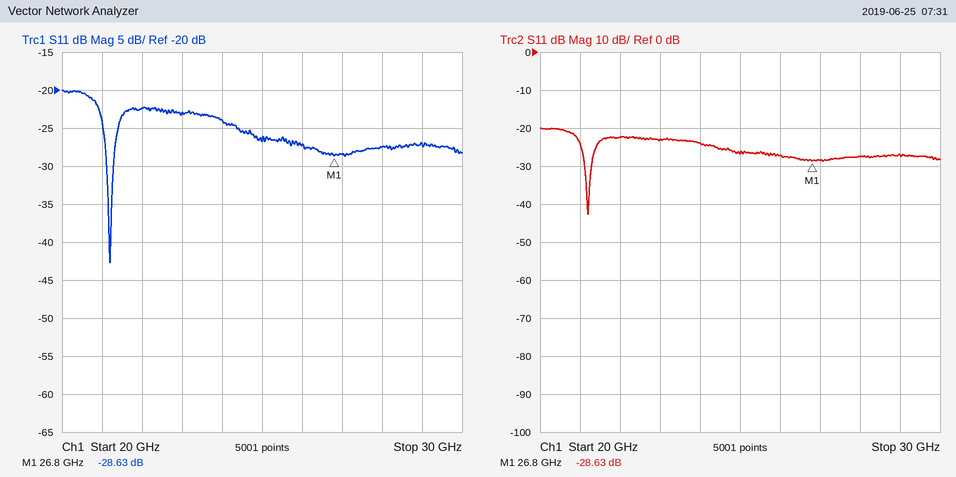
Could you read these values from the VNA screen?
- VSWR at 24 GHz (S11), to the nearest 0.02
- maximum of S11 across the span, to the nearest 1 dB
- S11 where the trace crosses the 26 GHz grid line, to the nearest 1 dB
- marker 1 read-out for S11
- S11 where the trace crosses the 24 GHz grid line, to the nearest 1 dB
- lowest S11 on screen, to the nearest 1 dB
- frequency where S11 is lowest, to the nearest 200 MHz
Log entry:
1.14
-20 dB
-27 dB
-28.63 dB
-24 dB
-43 dB
21.2 GHz
